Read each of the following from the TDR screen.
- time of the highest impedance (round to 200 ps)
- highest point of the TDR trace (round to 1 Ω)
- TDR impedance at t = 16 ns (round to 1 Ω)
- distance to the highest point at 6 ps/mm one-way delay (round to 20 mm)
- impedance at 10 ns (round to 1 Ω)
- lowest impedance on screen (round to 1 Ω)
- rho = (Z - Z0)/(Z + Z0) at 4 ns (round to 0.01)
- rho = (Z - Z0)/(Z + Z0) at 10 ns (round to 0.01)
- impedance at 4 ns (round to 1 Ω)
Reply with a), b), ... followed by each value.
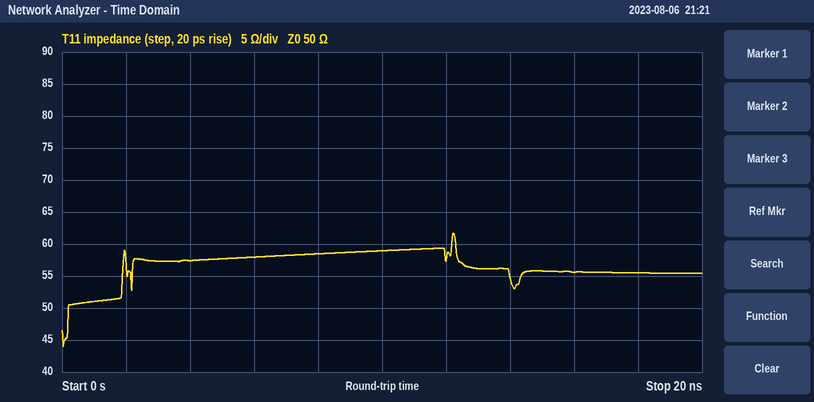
a) 12.2 ns
b) 62 Ω
c) 56 Ω
d) 1.02 m
e) 59 Ω
f) 44 Ω
g) +0.07
h) +0.08
i) 57 Ω
